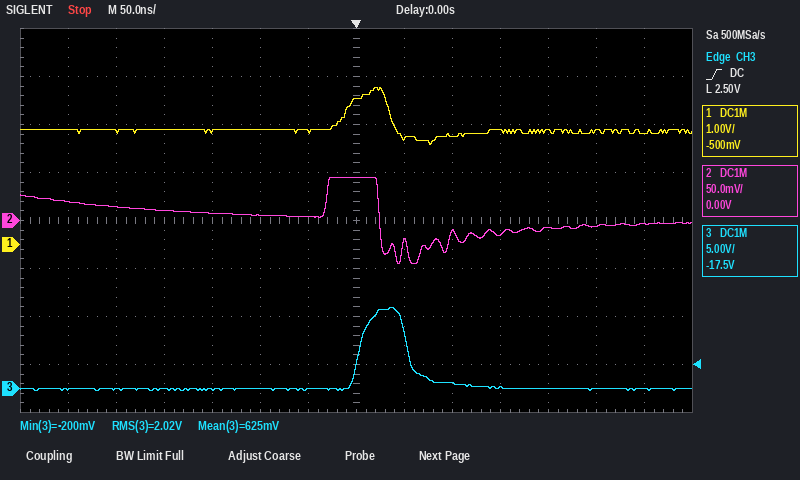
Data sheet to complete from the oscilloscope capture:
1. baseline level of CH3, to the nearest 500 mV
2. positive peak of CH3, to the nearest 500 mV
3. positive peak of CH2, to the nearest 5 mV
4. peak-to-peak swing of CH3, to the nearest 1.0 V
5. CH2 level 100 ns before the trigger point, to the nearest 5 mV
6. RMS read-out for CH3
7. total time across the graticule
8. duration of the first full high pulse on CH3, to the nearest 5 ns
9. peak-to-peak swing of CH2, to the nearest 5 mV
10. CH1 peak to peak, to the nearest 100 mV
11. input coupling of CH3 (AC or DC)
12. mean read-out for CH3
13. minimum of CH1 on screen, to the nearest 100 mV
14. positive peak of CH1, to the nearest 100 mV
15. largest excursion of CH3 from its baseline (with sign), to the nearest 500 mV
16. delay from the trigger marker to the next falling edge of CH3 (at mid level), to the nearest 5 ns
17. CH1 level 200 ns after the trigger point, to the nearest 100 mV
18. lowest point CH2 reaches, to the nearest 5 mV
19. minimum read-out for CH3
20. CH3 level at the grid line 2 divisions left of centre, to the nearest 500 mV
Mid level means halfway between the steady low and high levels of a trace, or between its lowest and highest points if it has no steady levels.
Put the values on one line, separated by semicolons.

0.0 V; 8.5 V; 45 mV; 9.0 V; 5 mV; 2.02 V; 700 ns; 50 ns; 90 mV; 1.2 V; DC; 625 mV; 2.1 V; 3.3 V; +8.5 V; 55 ns; 2.4 V; -45 mV; -200 mV; 0.0 V
